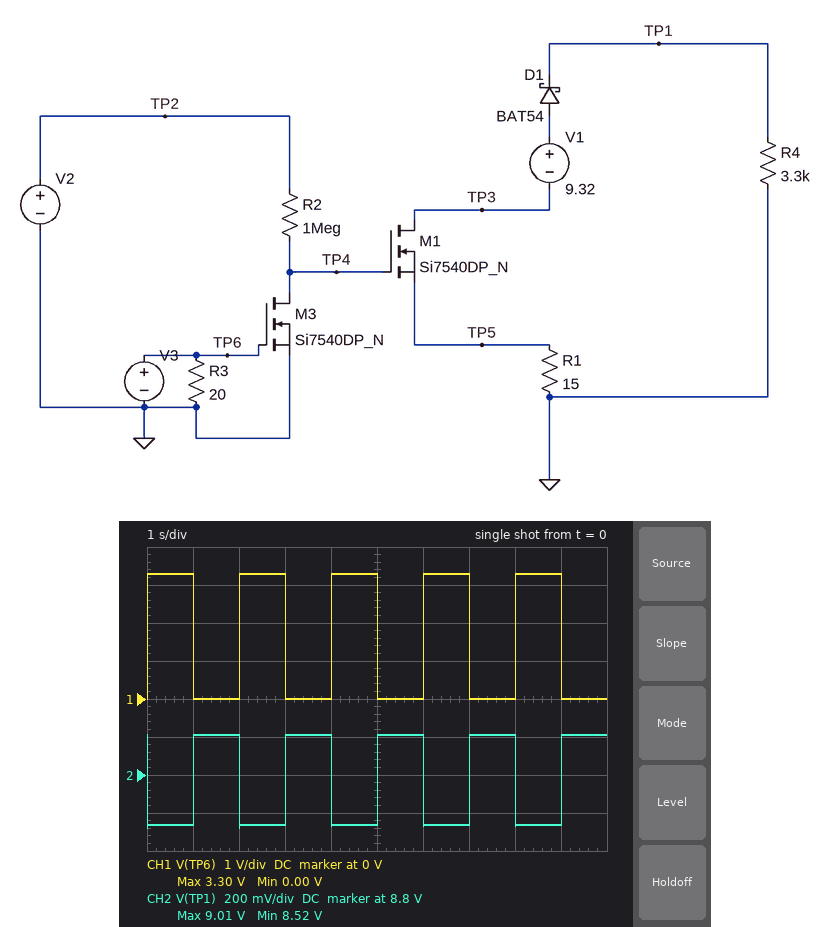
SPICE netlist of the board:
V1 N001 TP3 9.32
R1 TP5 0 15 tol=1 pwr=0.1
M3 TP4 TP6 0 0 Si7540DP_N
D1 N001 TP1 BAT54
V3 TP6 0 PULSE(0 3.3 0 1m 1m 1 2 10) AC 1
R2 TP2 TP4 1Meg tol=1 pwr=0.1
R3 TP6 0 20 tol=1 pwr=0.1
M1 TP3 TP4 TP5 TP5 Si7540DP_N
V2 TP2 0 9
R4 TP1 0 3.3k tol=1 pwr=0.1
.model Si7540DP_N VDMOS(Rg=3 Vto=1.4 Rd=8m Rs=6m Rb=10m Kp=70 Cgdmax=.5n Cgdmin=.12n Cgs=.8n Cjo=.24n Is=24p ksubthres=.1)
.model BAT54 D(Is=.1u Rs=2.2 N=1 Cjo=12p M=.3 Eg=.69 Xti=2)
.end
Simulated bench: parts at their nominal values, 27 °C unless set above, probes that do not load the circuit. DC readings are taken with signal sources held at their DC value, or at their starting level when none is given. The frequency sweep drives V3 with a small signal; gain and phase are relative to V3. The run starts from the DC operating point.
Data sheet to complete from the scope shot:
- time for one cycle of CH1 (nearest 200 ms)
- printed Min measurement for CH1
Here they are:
2.0 s
0.00 V
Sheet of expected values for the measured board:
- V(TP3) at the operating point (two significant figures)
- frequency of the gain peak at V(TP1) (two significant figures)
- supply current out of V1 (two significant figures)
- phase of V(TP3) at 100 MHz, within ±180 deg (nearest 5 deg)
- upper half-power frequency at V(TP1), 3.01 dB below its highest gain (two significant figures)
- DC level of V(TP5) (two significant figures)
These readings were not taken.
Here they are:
-41 mV
56 MHz
2.7 mA
-30 deg
140 MHz
-41 mV
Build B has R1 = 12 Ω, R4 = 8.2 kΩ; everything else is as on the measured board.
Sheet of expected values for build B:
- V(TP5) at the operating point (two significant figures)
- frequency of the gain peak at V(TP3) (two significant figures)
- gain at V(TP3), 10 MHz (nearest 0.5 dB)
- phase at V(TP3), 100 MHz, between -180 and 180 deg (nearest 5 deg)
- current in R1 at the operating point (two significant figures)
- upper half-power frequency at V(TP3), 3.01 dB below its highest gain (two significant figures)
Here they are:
-13 mV
61 MHz
-21.5 dB
-25 deg
1.1 mA
150 MHz
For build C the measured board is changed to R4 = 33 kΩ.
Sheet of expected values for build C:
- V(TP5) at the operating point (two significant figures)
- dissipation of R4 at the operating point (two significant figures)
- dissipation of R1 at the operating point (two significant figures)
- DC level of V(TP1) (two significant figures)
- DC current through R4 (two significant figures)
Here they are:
-4.1 mV
2.5 mW
1.1 µW
9.1 V
280 µA
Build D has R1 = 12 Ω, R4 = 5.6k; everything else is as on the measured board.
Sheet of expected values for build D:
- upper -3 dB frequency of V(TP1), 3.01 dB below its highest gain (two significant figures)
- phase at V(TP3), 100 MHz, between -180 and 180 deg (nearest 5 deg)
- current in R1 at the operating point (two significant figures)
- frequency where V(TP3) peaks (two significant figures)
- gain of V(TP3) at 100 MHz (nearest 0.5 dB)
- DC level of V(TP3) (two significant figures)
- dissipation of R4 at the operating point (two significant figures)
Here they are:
150 MHz
-25 deg
1.6 mA
61 MHz
-12.5 dB
-19 mV
15 mW
